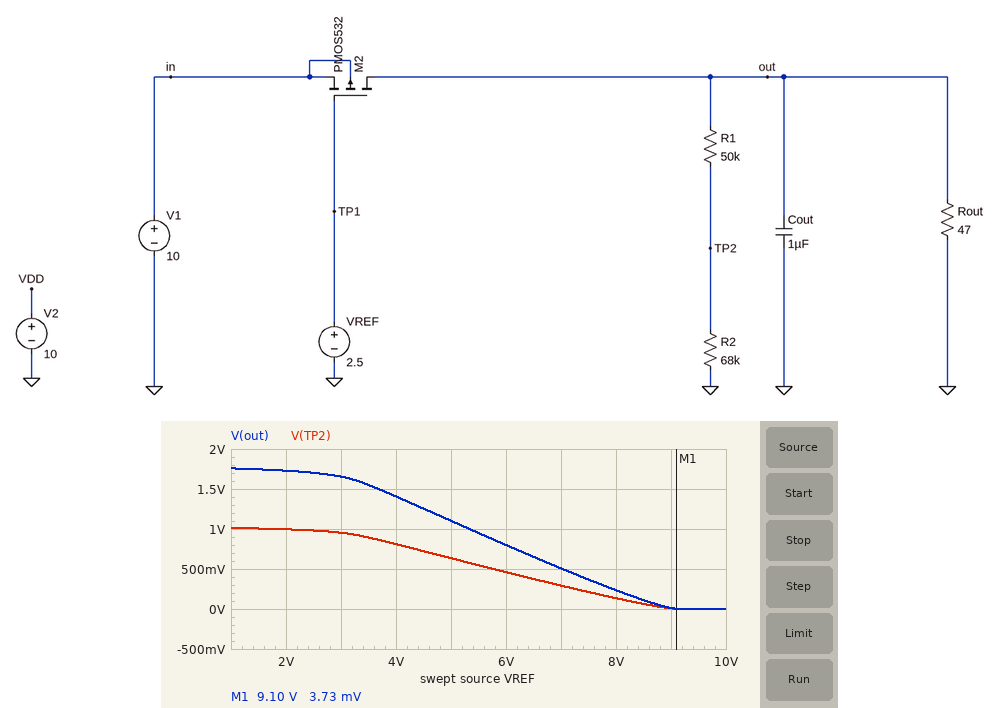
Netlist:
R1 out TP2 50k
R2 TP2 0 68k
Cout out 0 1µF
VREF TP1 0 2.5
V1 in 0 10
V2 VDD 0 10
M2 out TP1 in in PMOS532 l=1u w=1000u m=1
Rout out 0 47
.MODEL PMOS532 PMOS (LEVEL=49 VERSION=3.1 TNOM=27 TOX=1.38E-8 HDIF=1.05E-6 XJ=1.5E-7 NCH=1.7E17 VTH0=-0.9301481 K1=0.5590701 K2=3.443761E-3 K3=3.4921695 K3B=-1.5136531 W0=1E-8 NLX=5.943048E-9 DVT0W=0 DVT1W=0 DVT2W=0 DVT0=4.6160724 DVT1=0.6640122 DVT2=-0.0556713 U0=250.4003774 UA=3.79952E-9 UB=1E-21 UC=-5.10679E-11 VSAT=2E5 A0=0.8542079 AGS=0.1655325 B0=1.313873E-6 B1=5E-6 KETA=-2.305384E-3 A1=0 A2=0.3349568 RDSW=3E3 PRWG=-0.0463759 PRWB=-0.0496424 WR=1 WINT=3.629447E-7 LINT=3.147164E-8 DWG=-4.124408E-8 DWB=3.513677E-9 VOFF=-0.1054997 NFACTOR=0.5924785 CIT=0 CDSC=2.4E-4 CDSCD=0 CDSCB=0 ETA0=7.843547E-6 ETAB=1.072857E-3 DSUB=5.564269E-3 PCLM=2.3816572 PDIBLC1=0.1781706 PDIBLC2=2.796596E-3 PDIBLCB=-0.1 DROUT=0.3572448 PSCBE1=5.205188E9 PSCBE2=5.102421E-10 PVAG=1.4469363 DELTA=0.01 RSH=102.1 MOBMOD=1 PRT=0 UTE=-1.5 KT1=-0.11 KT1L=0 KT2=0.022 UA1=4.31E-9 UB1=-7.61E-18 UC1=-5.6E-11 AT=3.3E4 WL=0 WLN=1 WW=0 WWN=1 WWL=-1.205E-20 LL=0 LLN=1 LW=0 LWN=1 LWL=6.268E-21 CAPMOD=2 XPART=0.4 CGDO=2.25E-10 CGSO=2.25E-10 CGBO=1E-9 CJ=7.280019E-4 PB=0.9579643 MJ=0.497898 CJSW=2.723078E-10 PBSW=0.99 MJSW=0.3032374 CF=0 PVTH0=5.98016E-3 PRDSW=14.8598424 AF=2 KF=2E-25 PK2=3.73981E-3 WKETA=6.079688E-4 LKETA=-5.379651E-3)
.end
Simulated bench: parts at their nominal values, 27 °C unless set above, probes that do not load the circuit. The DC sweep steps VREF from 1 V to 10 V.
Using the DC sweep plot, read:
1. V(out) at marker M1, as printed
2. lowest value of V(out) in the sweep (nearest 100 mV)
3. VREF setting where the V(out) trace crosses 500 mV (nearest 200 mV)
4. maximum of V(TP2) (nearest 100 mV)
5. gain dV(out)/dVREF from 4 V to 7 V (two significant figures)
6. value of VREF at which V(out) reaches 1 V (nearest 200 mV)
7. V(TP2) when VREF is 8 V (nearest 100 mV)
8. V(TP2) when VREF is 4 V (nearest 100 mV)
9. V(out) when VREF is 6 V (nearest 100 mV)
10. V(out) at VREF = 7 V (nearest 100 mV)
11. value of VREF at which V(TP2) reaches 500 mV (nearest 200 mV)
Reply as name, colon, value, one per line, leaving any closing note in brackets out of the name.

V(out) at marker M1, as printed: 3.73 mV
lowest value of V(out) in the sweep: 0 V
VREF setting where the V(out) trace crosses 500 mV: 7.0 V
maximum of V(TP2): 1.0 V
gain dV(out)/dVREF from 4 V to 7 V: -0.30 V/V
value of VREF at which V(out) reaches 1 V: 5.4 V
V(TP2) when VREF is 8 V: 100 mV
V(TP2) when VREF is 4 V: 800 mV
V(out) when VREF is 6 V: 800 mV
V(out) at VREF = 7 V: 500 mV
value of VREF at which V(TP2) reaches 500 mV: 5.8 V
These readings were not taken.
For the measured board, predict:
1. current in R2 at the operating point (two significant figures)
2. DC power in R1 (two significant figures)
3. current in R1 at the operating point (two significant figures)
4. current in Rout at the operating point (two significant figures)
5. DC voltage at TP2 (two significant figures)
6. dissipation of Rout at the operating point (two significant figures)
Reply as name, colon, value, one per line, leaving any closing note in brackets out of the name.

current in R2 at the operating point: 14 µA
DC power in R1: 10 µW
current in R1 at the operating point: 14 µA
current in Rout at the operating point: 36 mA
DC voltage at TP2: 980 mV
dissipation of Rout at the operating point: 62 mW
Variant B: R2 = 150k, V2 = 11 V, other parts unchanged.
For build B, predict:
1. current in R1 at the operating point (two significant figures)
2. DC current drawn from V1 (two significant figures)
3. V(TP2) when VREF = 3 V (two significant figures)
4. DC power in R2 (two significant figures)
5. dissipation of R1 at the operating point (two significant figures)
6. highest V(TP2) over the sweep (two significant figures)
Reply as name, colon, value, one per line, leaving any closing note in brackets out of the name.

current in R1 at the operating point: 8.5 µA
DC current drawn from V1: 36 mA
V(TP2) when VREF = 3 V: 1.2 V
DC power in R2: 11 µW
dissipation of R1 at the operating point: 3.6 µW
highest V(TP2) over the sweep: 1.3 V
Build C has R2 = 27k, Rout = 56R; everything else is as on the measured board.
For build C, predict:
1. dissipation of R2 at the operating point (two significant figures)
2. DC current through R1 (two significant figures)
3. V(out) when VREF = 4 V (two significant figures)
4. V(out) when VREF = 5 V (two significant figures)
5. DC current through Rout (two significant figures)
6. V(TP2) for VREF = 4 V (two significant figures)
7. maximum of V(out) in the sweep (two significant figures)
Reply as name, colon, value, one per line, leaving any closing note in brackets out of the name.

dissipation of R2 at the operating point: 18 µW
DC current through R1: 26 µA
V(out) when VREF = 4 V: 1.7 V
V(out) when VREF = 5 V: 1.3 V
DC current through Rout: 35 mA
V(TP2) for VREF = 4 V: 590 mV
maximum of V(out) in the sweep: 2.0 V
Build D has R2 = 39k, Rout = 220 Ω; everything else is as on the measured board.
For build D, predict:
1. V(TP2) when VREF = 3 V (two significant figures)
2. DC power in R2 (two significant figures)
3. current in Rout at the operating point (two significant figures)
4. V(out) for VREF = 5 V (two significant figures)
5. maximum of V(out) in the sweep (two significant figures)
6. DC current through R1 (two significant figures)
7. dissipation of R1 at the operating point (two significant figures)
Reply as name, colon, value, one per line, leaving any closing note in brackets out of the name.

V(TP2) when VREF = 3 V: 2.2 V
DC power in R2: 120 µW
current in Rout at the operating point: 23 mA
V(out) for VREF = 5 V: 4.8 V
maximum of V(out) in the sweep: 5.0 V
DC current through R1: 56 µA
dissipation of R1 at the operating point: 160 µW
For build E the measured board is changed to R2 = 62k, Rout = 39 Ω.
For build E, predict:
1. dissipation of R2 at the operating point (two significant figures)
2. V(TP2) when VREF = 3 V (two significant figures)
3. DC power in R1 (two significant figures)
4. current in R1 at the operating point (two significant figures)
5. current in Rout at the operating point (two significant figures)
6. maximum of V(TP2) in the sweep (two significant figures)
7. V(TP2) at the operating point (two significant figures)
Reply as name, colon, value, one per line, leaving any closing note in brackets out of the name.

dissipation of R2 at the operating point: 10 µW
V(TP2) when VREF = 3 V: 770 mV
DC power in R1: 8.3 µW
current in R1 at the operating point: 13 µA
current in Rout at the operating point: 37 mA
maximum of V(TP2) in the sweep: 830 mV
V(TP2) at the operating point: 800 mV
